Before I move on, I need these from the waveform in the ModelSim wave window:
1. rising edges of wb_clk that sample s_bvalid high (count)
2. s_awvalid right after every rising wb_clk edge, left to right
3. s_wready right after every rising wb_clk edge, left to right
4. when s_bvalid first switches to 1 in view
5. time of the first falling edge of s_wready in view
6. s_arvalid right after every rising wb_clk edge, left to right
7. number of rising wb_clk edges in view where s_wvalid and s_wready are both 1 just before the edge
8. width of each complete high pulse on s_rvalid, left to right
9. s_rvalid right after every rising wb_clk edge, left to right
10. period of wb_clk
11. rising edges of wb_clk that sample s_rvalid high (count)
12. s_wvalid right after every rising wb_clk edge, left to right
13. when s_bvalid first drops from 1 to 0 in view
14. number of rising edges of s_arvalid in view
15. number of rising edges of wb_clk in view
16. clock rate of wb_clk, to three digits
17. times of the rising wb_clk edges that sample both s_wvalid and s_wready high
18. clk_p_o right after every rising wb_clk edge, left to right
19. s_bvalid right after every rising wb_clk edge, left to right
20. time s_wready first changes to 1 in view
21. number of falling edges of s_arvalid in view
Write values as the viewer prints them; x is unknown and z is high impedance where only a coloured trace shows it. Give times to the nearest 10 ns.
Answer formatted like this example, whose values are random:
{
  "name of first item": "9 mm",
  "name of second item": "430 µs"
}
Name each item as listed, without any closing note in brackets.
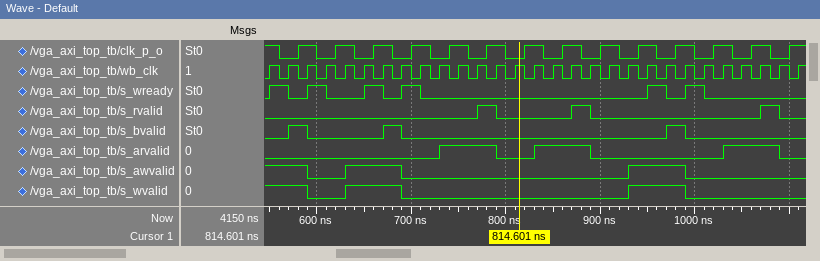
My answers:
{
  "rising edges of wb_clk that sample s_bvalid high": "3",
  "s_awvalid right after every rising wb_clk edge, left to right": "1 1 0 0 1 1 1 0 0 0 0 0 0 0 0 0 0 0 0 1 1 1 0 0 0 0 0 0 0",
  "s_wready right after every rising wb_clk edge, left to right": "1 0 1 0 0 1 0 1 0 0 0 0 0 0 0 0 0 0 0 0 1 0 1 0 0 0 0 0 0",
  "when s_bvalid first switches to 1 in view": "570 ns",
  "time of the first falling edge of s_wready in view": "570 ns",
  "s_arvalid right after every rising wb_clk edge, left to right": "0 0 0 0 0 0 0 0 0 1 1 1 0 0 1 1 1 0 0 0 0 0 0 0 1 1 1 0 0",
  "number of rising wb_clk edges in view where s_wvalid and s_wready are both 1 just before the edge": "3",
  "width of each complete high pulse on s_rvalid, left to right": "20 ns, 20 ns, 20 ns",
  "s_rvalid right after every rising wb_clk edge, left to right": "0 0 0 0 0 0 0 0 0 0 0 1 0 0 0 0 1 0 0 0 0 0 0 0 0 0 1 0 0",
  "period of wb_clk": "20 ns",
  "rising edges of wb_clk that sample s_rvalid high": "3",
  "s_wvalid right after every rising wb_clk edge, left to right": "1 1 0 0 1 1 1 0 0 0 0 0 0 0 0 0 0 0 0 1 1 1 0 0 0 0 0 0 0",
  "when s_bvalid first drops from 1 to 0 in view": "590 ns",
  "number of rising edges of s_arvalid in view": "3",
  "number of rising edges of wb_clk in view": "29",
  "clock rate of wb_clk, to three digits": "50.0 MHz",
  "times of the rising wb_clk edges that sample both s_wvalid and s_wready high": "570 ns, 670 ns, 970 ns",
  "clk_p_o right after every rising wb_clk edge, left to right": "1 0 1 0 1 0 1 0 1 0 1 0 1 0 1 0 1 0 1 0 1 0 1 0 1 0 1 0 1",
  "s_bvalid right after every rising wb_clk edge, left to right": "0 1 0 0 0 0 1 0 0 0 0 0 0 0 0 0 0 0 0 0 0 1 0 0 0 0 0 0 0",
  "time s_wready first changes to 1 in view": "550 ns",
  "number of falling edges of s_arvalid in view": "3"
}
